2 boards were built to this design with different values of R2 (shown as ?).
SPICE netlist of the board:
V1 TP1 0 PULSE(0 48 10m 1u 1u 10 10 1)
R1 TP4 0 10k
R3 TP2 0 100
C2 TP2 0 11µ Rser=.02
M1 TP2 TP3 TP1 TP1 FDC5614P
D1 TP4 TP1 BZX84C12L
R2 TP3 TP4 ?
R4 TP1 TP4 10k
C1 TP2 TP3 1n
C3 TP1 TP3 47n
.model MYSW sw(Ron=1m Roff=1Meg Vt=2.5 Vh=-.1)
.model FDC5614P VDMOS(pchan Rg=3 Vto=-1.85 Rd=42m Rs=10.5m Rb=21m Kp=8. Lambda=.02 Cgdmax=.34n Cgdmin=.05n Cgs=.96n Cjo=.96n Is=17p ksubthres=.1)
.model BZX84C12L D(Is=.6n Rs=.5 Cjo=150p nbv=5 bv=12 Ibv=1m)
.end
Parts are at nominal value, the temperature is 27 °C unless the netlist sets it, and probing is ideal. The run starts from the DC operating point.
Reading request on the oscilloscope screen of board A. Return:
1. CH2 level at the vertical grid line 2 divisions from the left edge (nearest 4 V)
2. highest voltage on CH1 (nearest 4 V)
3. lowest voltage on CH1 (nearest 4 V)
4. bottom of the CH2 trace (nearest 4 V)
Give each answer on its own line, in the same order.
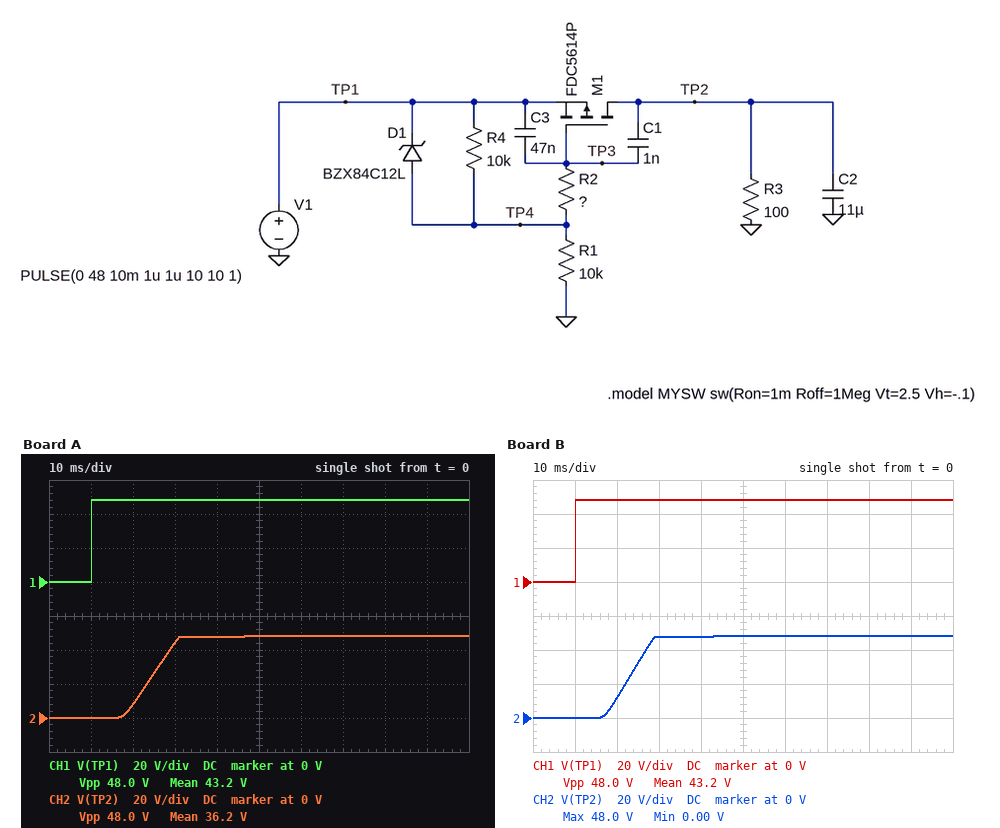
8 V
48 V
0 V
0 V
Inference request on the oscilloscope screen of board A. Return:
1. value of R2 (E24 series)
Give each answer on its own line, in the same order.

2 MΩ
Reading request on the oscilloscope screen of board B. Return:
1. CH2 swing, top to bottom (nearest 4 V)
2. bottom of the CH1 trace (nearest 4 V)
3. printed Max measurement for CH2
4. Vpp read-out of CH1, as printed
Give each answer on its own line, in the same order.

48 V
0 V
48.0 V
48.0 V
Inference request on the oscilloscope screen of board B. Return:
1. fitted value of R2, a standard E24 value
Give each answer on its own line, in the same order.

1.8 MΩ
